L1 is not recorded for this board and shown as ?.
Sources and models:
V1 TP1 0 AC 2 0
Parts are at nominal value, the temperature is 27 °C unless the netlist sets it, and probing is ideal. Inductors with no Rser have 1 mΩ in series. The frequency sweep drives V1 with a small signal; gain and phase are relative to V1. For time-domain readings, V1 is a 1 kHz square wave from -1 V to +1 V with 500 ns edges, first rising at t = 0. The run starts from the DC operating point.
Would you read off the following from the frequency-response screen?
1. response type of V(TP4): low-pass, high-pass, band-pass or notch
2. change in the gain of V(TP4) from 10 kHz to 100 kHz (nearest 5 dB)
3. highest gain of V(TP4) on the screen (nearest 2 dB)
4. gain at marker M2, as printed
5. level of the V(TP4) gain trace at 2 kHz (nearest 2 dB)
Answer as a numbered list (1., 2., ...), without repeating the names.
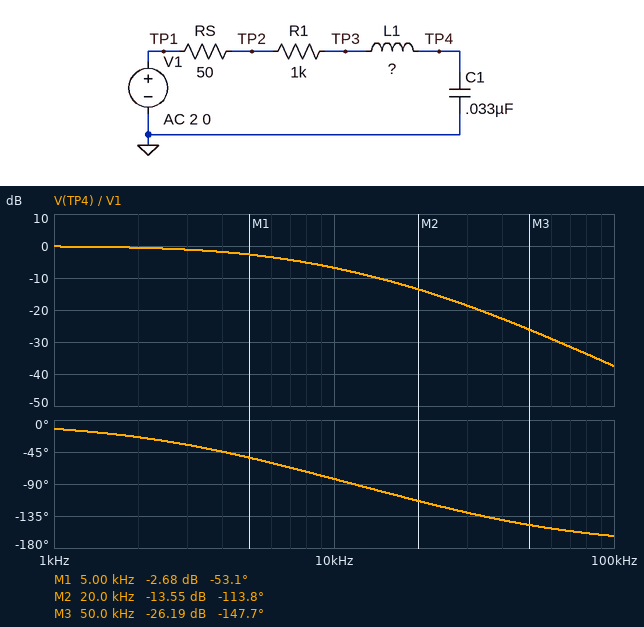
1. low-pass
2. -30 dB
3. 0 dB
4. -13.55 dB
5. 0 dB
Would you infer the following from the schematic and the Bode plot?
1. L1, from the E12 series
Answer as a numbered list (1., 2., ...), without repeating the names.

1. 5.6 mH
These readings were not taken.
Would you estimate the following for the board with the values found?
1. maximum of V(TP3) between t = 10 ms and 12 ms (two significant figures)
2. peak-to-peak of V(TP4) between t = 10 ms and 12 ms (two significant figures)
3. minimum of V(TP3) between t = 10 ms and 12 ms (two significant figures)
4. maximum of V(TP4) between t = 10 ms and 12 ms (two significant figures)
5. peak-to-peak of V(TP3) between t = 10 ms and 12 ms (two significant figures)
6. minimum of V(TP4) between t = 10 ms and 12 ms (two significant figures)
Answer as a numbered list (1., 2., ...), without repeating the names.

1. 1.0 V
2. 2.0 V
3. -1.0 V
4. 1.0 V
5. 2.0 V
6. -1.0 V
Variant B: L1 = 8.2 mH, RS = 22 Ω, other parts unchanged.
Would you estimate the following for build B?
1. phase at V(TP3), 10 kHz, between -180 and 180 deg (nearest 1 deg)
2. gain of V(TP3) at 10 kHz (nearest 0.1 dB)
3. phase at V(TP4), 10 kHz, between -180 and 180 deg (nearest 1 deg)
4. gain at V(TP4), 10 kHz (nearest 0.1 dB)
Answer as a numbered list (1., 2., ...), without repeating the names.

1. 88 deg
2. -29.8 dB
3. -92 deg
4. -6.5 dB
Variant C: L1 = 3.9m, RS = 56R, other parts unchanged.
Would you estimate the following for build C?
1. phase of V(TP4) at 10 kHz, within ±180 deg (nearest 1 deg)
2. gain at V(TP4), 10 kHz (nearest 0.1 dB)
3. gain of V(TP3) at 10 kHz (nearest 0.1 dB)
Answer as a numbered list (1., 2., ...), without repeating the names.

1. -77 deg
2. -7.0 dB
3. -13.2 dB
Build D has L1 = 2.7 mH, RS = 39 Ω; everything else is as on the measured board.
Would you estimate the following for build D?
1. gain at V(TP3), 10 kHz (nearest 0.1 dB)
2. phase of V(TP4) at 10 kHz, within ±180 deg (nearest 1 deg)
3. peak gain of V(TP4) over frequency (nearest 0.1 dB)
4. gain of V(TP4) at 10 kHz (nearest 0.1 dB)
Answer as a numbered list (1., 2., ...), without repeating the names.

1. -10.8 dB
2. -73 deg
3. 0 dB
4. -7.0 dB
